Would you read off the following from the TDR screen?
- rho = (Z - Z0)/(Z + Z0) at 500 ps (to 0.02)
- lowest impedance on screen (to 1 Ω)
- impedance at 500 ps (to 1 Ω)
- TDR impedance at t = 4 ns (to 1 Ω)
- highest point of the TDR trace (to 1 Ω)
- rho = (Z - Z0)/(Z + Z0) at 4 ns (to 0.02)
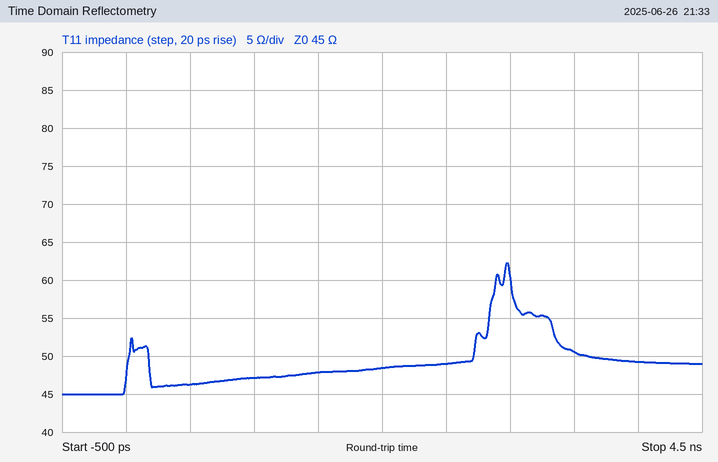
+0.02
45 Ω
46 Ω
49 Ω
62 Ω
+0.04
